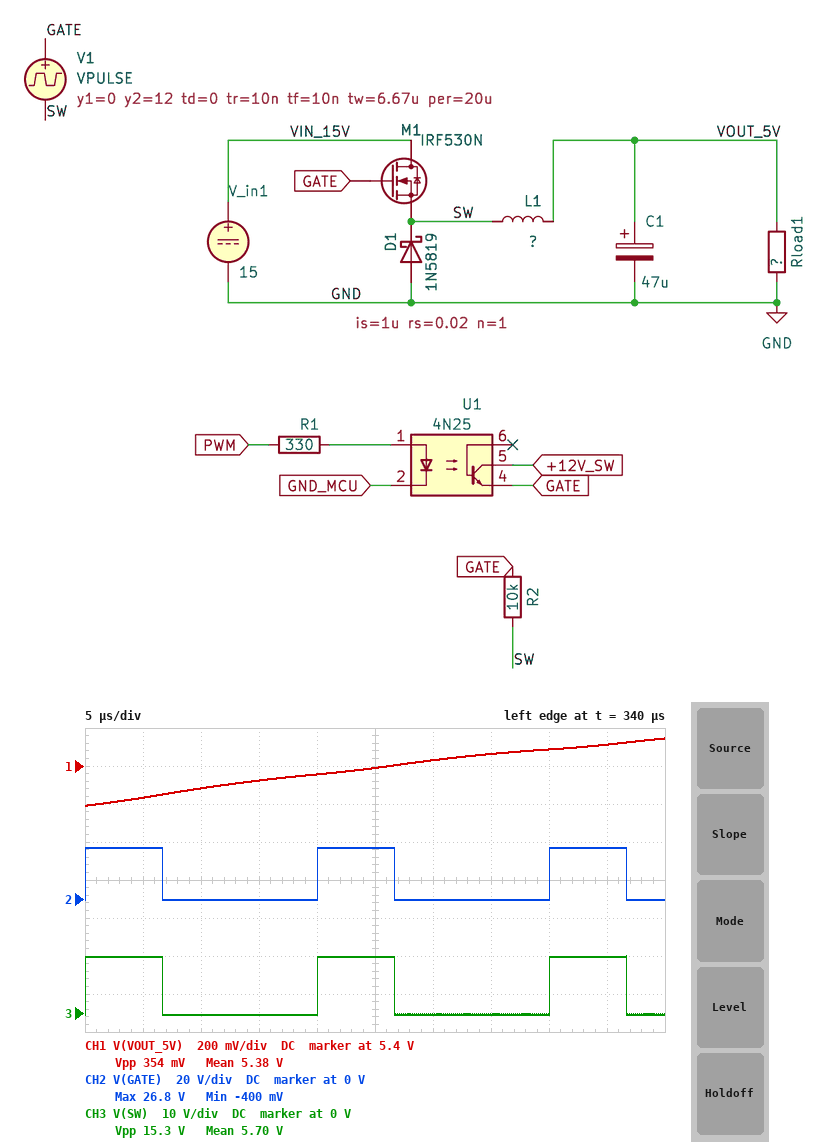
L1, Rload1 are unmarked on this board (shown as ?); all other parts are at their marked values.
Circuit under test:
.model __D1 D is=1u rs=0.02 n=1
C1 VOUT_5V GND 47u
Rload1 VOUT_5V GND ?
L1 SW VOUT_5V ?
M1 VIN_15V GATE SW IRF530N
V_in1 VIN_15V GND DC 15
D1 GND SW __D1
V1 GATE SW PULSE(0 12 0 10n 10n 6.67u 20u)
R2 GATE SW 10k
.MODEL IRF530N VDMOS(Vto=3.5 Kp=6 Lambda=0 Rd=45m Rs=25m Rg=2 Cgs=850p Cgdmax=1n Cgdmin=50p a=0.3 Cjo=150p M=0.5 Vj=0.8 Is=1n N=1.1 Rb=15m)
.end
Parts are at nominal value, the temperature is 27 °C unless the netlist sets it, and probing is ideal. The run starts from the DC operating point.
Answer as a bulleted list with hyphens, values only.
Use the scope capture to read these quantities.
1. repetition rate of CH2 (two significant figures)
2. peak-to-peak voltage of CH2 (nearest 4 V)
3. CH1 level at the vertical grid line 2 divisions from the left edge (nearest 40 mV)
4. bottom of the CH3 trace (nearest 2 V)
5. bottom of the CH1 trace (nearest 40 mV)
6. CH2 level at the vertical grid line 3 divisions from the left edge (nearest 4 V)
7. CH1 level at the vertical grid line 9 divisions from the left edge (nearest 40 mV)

- 50 kHz
- 28 V
- 5.28 V
- 0 V
- 5.20 V
- 0 V
- 5.52 V
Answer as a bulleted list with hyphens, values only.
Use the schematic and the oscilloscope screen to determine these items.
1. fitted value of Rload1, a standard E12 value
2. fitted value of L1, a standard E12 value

- 3.3 Ω
- 390 µH
